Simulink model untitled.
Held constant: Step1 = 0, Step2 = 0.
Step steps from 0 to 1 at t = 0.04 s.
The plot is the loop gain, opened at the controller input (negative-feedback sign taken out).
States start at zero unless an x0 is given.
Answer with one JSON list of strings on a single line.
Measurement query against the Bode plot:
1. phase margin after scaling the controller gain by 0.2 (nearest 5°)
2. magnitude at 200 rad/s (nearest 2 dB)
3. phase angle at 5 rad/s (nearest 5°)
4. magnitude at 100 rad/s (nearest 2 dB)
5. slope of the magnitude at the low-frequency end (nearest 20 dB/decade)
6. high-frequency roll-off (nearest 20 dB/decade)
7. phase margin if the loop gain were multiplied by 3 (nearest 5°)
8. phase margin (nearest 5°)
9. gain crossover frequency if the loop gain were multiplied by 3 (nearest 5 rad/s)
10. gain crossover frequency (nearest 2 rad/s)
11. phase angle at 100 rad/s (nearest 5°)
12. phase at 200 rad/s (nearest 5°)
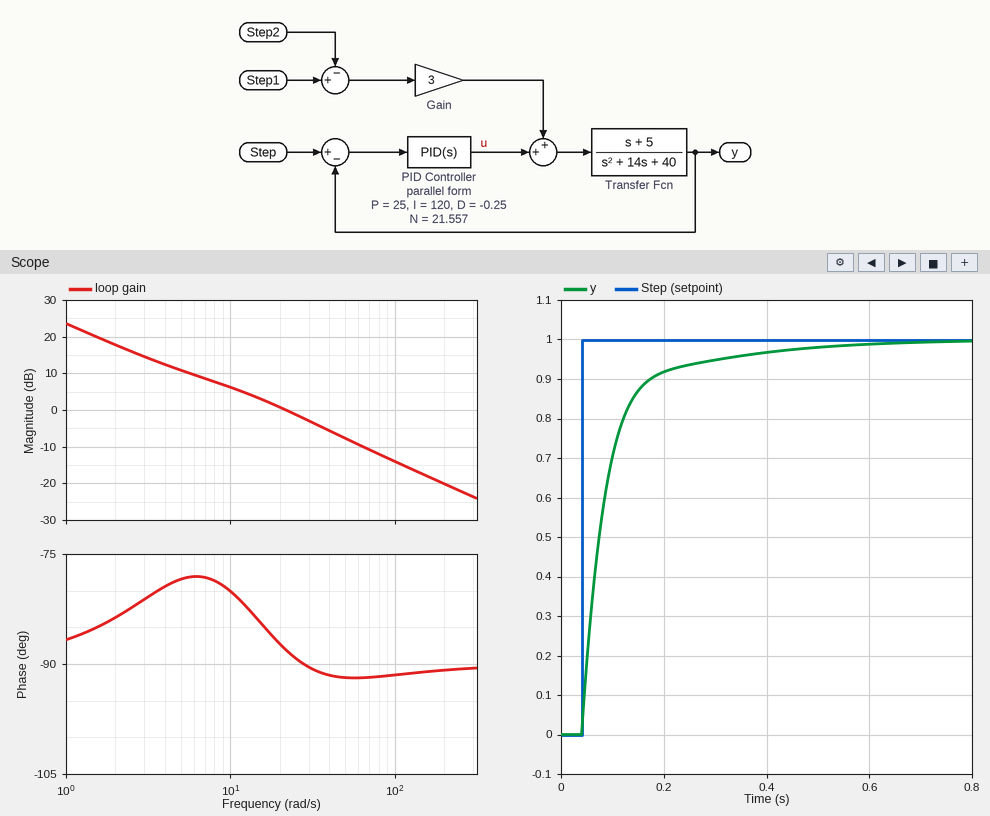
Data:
["100°", "-20 dB", "-80°", "-14 dB", "-20 dB/decade", "-20 dB/decade", "90°", "90°", "60 rad/s", "22 rad/s", "-90°", "-90°"]
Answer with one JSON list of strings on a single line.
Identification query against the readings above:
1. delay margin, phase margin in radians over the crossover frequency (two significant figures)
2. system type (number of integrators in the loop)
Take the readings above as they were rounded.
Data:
["0.071 s", "1"]
